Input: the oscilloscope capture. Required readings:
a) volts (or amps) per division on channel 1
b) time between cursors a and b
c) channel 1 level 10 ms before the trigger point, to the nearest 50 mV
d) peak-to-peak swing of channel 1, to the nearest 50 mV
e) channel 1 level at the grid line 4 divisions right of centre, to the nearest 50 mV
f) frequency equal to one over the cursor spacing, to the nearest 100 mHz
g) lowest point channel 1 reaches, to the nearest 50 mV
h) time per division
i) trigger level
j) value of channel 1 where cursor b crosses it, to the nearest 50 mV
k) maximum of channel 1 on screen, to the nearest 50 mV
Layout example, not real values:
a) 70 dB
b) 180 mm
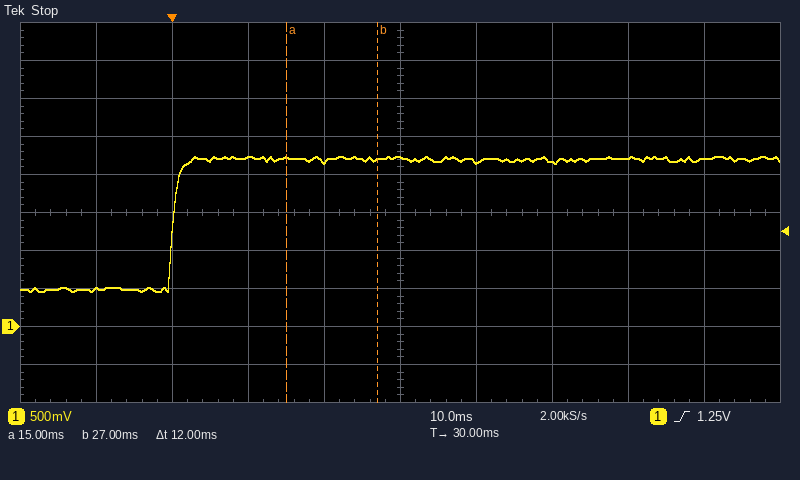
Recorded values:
a) 500 mV
b) 12 ms
c) 500 mV
d) 1.80 V
e) 2.20 V
f) 83.3 Hz
g) 450 mV
h) 10 ms
i) 1.25 V
j) 2.20 V
k) 2.25 V
